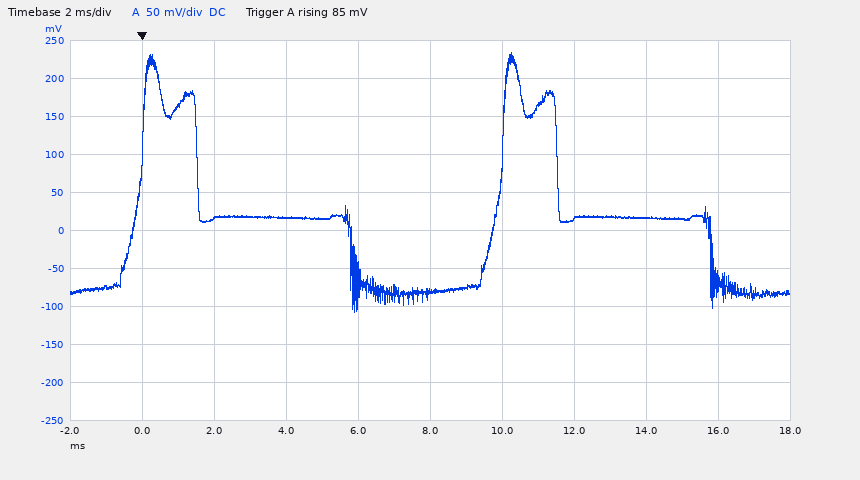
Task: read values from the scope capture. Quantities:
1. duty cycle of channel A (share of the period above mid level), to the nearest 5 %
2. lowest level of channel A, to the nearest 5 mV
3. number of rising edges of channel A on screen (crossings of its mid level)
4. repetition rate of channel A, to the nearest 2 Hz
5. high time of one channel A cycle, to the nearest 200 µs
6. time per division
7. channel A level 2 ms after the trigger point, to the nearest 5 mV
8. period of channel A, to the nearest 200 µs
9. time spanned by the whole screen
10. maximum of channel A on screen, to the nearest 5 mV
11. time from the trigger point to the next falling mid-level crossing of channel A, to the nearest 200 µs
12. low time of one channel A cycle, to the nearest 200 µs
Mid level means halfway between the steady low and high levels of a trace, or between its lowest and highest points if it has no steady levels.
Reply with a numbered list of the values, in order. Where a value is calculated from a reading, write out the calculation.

1. 1.6 ms / 10.0 ms ≈ 16.0 %, so 15 % to the nearest 5 %
2. -110 mV
3. 2
4. 1 / 10.0 ms ≈ 100 Hz
5. 1.6 ms
6. 2 ms
7. 15 mV
8. 10.0 ms
9. 20 ms
10. 235 mV
11. 1.6 ms
12. 8.4 ms
